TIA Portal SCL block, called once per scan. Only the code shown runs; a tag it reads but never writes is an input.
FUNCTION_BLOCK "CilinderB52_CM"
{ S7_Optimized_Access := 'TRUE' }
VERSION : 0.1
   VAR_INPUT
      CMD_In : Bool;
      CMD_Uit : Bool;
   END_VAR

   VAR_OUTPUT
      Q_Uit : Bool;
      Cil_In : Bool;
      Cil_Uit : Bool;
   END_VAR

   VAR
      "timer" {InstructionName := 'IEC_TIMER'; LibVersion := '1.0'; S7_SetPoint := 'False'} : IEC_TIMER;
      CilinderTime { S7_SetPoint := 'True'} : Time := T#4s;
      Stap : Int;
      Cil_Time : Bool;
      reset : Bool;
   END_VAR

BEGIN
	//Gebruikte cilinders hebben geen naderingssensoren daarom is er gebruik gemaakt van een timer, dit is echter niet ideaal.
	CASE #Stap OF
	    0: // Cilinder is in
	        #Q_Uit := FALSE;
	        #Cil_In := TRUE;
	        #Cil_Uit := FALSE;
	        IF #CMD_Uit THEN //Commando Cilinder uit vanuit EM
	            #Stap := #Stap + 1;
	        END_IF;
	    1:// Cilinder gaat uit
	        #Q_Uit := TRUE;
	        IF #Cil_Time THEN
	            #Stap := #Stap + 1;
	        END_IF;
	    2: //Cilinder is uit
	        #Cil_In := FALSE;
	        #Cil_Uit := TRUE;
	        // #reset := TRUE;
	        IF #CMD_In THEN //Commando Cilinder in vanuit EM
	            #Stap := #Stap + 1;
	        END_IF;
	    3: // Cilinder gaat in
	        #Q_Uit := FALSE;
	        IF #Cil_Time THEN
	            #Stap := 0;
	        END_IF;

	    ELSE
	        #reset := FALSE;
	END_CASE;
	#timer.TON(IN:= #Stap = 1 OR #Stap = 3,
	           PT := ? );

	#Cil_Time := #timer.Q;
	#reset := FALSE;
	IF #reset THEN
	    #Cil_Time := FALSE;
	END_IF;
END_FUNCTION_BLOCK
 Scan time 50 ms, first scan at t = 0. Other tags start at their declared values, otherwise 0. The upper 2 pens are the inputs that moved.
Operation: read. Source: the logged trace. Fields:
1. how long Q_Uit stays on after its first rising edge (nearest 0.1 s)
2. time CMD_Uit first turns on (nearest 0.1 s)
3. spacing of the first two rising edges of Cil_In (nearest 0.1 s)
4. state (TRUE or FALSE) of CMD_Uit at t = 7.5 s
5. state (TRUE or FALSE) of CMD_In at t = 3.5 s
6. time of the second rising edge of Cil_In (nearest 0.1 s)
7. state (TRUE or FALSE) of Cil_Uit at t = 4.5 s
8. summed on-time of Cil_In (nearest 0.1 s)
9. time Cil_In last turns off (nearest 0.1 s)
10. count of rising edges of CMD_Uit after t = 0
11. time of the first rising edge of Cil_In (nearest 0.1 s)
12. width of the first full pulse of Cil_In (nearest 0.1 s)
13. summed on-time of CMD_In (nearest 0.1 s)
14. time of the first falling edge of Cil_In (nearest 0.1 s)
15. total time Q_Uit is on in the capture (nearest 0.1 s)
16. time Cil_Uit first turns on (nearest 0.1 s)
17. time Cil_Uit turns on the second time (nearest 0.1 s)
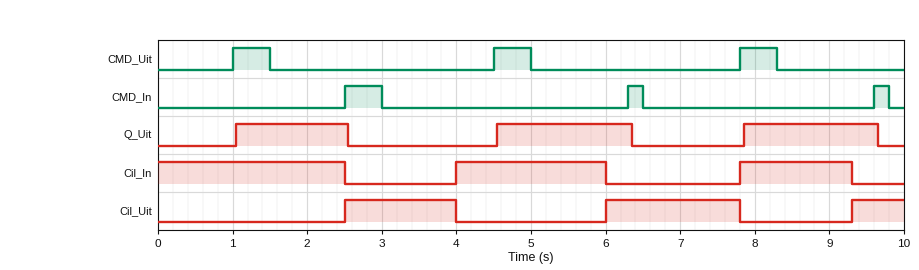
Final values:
1.5 s
1.0 s
3.8 s
FALSE
FALSE
7.8 s
FALSE
6.0 s
9.3 s
3
4.0 s
2.0 s
0.9 s
2.5 s
5.1 s
2.5 s
6.0 s
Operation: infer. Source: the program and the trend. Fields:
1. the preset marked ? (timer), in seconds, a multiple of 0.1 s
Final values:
1.4 s
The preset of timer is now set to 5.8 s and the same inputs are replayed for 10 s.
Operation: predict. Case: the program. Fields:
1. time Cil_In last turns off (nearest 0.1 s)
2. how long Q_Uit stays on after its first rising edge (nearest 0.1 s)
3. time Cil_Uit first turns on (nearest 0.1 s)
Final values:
6.9 s
8.6 s
6.9 s
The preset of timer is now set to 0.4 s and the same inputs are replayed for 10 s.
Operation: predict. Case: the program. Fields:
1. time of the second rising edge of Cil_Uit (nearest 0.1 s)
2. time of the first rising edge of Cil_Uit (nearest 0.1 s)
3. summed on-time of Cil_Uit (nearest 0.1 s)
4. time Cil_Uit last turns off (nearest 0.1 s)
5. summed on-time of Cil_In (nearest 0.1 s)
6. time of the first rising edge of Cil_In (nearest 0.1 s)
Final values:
5.0 s
1.5 s
5.0 s
6.8 s
5.0 s
3.0 s
